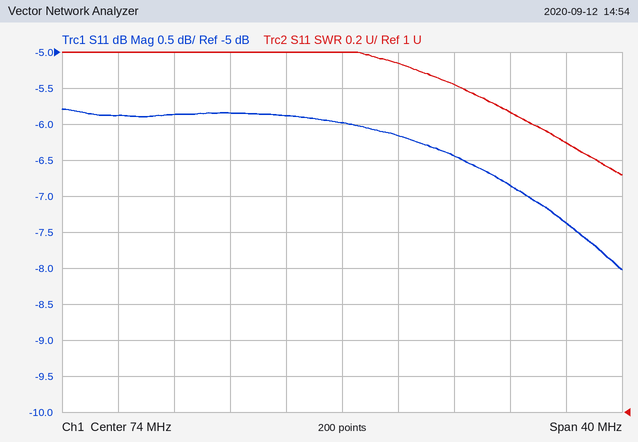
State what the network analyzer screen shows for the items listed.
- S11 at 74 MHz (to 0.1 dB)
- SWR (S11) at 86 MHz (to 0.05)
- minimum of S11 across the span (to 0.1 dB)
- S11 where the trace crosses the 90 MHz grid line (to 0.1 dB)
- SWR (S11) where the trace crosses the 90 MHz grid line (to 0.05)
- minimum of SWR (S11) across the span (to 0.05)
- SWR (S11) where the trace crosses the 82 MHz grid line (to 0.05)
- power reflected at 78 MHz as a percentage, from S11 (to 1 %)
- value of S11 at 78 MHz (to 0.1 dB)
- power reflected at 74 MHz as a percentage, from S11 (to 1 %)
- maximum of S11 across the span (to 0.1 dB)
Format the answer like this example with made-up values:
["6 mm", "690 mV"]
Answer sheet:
["-6.0 dB", "2.65", "-8.0 dB", "-7.4 dB", "2.50", "2.30", "2.80", "24 %", "-6.2 dB", "25 %", "-5.8 dB"]
